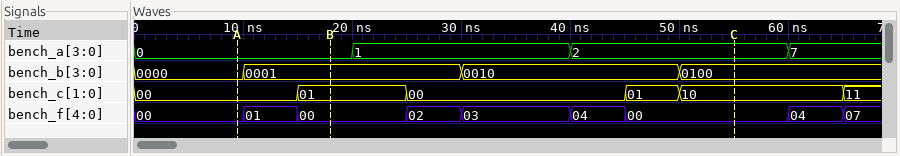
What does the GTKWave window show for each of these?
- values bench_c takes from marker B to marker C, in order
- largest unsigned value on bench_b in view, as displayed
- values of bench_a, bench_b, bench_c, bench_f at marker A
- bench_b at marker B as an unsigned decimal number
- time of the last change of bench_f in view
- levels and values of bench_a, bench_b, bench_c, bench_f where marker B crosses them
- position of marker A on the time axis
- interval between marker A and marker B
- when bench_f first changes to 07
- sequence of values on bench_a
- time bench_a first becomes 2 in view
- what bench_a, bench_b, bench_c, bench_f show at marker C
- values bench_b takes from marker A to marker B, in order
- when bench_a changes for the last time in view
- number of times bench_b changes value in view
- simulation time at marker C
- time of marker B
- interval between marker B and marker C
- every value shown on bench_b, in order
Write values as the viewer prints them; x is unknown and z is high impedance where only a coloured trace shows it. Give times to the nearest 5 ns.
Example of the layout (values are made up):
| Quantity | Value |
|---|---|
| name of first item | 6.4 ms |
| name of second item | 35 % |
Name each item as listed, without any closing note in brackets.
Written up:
| Quantity | Value |
|---|---|
| values bench_c takes from marker B to marker C, in order | 01, 00, 01, 10 |
| largest unsigned value on bench_b in view, as displayed | 0100 |
| values of bench_a, bench_b, bench_c, bench_f at marker A | bench_a=0, bench_b=0000, bench_c=00, bench_f=00 |
| bench_b at marker B as an unsigned decimal number | 1 |
| time of the last change of bench_f in view | 65 ns |
| levels and values of bench_a, bench_b, bench_c, bench_f where marker B crosses them | bench_a=0, bench_b=0001, bench_c=01, bench_f=00 |
| position of marker A on the time axis | 10 ns |
| interval between marker A and marker B | 10 ns |
| when bench_f first changes to 07 | 65 ns |
| sequence of values on bench_a | 0, 1, 2, 7 |
| time bench_a first becomes 2 in view | 40 ns |
| what bench_a, bench_b, bench_c, bench_f show at marker C | bench_a=2, bench_b=0100, bench_c=10, bench_f=00 |
| values bench_b takes from marker A to marker B, in order | 0000, 0001 |
| when bench_a changes for the last time in view | 60 ns |
| number of times bench_b changes value in view | 3 |
| simulation time at marker C | 55 ns |
| time of marker B | 20 ns |
| interval between marker B and marker C | 35 ns |
| every value shown on bench_b, in order | 0000, 0001, 0010, 0100 |
